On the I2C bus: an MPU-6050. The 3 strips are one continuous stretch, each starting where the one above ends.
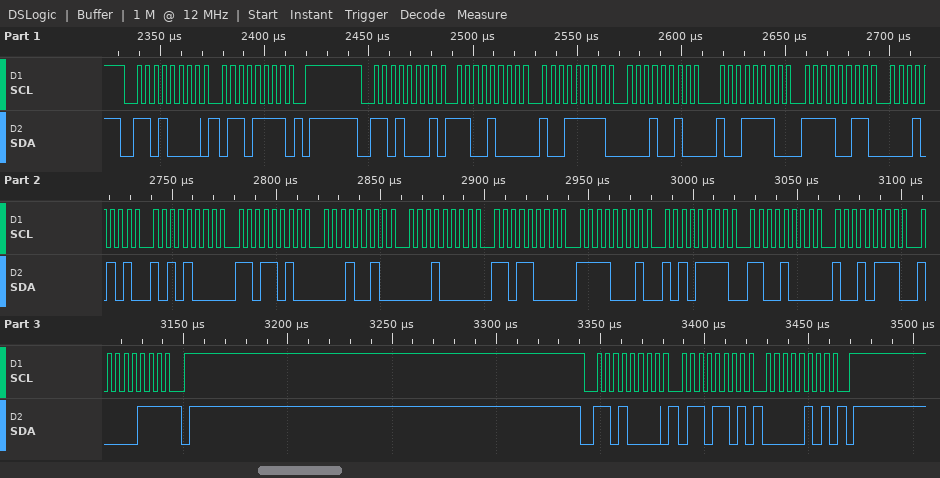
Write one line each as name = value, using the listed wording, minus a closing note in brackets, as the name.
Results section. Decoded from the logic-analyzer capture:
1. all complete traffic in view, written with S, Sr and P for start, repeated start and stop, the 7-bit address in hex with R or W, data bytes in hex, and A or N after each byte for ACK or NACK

all complete traffic in view, written with S, Sr and P for start, repeated start and stop, the 7-bit address in hex with R or W, data bytes in hex, and A or N after each byte for ACK or NACK = S 68W A 6F A P S 68R A C8 A 9F A 12 A 9E A F3 A 15 A A8 A DA A 12 A 10 A D8 A F1 A AF A C8 A 97 A 87 N P S 68W A 6D A 05 A P
